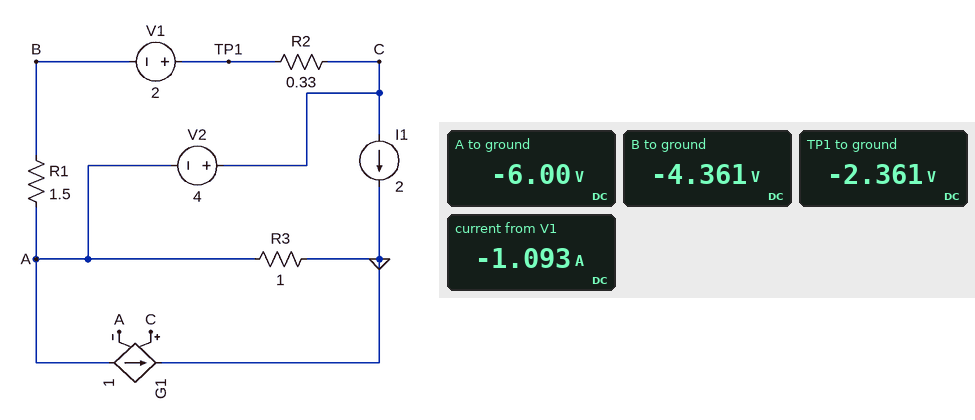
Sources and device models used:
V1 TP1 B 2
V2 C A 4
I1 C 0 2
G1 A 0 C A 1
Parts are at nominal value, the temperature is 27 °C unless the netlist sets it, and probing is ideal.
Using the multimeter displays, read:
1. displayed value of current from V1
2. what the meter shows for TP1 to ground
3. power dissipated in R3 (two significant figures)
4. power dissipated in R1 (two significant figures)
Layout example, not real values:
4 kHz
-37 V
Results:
-1.093 A
-2.361 V
36 W
1.8 W
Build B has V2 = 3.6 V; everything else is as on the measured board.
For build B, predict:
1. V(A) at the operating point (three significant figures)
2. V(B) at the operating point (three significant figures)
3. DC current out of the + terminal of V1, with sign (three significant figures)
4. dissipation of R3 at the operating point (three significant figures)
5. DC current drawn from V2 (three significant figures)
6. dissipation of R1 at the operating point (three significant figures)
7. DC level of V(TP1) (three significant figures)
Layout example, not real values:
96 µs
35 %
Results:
-5.60 V
-4.29 V
-874 mA
31.4 W
2.87 A
1.15 W
-2.29 V
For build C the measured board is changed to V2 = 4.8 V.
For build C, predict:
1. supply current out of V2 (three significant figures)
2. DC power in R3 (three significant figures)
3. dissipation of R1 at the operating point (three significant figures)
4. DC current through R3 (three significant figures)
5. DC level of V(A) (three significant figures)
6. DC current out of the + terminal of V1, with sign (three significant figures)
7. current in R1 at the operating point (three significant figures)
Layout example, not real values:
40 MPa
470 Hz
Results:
3.53 A
46.2 W
3.51 W
6.80 A
-6.80 V
-1.53 A
1.53 A
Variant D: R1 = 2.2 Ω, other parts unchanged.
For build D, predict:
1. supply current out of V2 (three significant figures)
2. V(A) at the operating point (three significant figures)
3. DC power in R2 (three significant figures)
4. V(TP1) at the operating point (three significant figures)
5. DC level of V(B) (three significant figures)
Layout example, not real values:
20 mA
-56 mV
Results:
2.79 A
-6.00 V
206 mW
-2.26 V
-4.26 V
